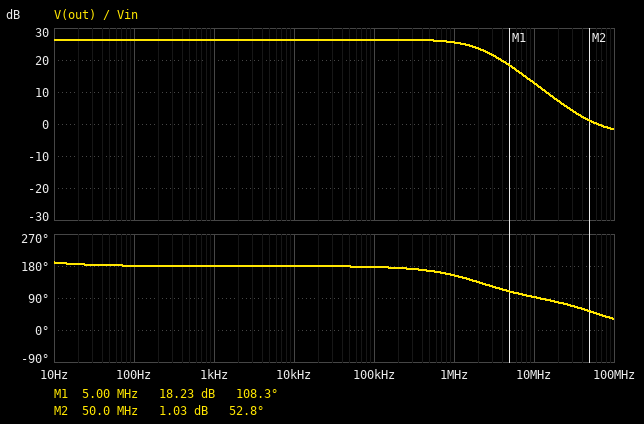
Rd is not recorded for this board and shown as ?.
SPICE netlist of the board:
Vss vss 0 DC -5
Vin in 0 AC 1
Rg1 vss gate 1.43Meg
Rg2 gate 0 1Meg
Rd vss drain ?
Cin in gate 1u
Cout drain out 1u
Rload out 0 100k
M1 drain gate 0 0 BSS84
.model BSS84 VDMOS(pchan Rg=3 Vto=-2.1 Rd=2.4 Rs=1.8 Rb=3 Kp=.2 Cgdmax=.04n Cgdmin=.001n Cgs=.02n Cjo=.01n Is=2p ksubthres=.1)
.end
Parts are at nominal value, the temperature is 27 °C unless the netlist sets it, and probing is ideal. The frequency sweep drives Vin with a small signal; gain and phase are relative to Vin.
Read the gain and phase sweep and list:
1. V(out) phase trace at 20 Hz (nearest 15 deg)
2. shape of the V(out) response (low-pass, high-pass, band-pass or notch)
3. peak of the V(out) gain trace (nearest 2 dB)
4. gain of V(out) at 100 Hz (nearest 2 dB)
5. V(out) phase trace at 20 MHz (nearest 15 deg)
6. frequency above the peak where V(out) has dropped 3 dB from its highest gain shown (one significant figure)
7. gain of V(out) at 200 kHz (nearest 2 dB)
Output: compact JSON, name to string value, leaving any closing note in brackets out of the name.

{"V(out) phase trace at 20 Hz": "180 deg", "shape of the V(out) response": "low-pass", "peak of the V(out) gain trace": "26 dB", "gain of V(out) at 100 Hz": "26 dB", "V(out) phase trace at 20 MHz": "75 deg", "frequency above the peak where V(out) has dropped 3 dB from its highest gain shown": "2 MHz", "gain of V(out) at 200 kHz": "26 dB"}
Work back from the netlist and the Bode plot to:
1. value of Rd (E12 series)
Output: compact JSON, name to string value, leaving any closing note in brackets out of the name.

{"value of Rd": "5.6 kΩ"}
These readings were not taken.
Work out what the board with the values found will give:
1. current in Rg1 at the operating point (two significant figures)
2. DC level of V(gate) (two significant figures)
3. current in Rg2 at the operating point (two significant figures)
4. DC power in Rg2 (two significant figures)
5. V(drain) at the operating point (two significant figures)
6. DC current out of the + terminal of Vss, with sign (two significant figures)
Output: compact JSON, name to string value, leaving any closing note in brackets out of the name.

{"current in Rg1 at the operating point": "2.1 µA", "DC level of V(gate)": "-2.1 V", "current in Rg2 at the operating point": "2.1 µA", "DC power in Rg2": "4.2 µW", "V(drain) at the operating point": "-3.6 V", "DC current out of the + terminal of Vss, with sign": "-250 µA"}
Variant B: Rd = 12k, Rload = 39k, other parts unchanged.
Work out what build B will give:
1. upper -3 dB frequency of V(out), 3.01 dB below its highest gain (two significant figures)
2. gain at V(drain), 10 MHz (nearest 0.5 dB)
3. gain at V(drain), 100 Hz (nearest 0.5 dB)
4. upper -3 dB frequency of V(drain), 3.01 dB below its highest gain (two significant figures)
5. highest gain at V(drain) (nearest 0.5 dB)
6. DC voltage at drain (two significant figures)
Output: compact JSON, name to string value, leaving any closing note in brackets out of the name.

{"upper -3 dB frequency of V(out), 3.01 dB below its highest gain": "550 kHz", "gain at V(drain), 10 MHz": "6.5 dB", "gain at V(drain), 100 Hz": "31.0 dB", "upper -3 dB frequency of V(drain), 3.01 dB below its highest gain": "300 kHz", "highest gain at V(drain)": "33.0 dB", "DC voltage at drain": "-2.0 V"}
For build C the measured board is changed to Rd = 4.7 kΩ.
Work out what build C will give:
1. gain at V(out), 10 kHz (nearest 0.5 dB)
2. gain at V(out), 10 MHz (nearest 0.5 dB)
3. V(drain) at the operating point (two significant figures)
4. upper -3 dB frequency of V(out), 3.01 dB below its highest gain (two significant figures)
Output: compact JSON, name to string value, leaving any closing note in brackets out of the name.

{"gain at V(out), 10 kHz": "25.0 dB", "gain at V(out), 10 MHz": "13.5 dB", "V(drain) at the operating point": "-3.8 V", "upper -3 dB frequency of V(out), 3.01 dB below its highest gain": "2.7 MHz"}
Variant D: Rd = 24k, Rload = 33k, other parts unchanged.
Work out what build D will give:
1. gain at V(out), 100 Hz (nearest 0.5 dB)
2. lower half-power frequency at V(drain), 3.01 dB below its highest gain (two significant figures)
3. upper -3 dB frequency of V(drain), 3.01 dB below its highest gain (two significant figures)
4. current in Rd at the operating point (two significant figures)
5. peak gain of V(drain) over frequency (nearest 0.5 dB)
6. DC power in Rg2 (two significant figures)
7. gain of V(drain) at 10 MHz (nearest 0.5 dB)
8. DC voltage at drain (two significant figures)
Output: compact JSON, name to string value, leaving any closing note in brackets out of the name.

{"gain at V(out), 100 Hz": "-5.5 dB", "lower half-power frequency at V(drain), 3.01 dB below its highest gain": "4.1 MHz", "upper -3 dB frequency of V(drain), 3.01 dB below its highest gain": "1.4 GHz", "current in Rd at the operating point": "210 µA", "peak gain of V(drain) over frequency": "-2.0 dB", "DC power in Rg2": "4.2 µW", "gain of V(drain) at 10 MHz": "-4.0 dB", "DC voltage at drain": "-30 mV"}
